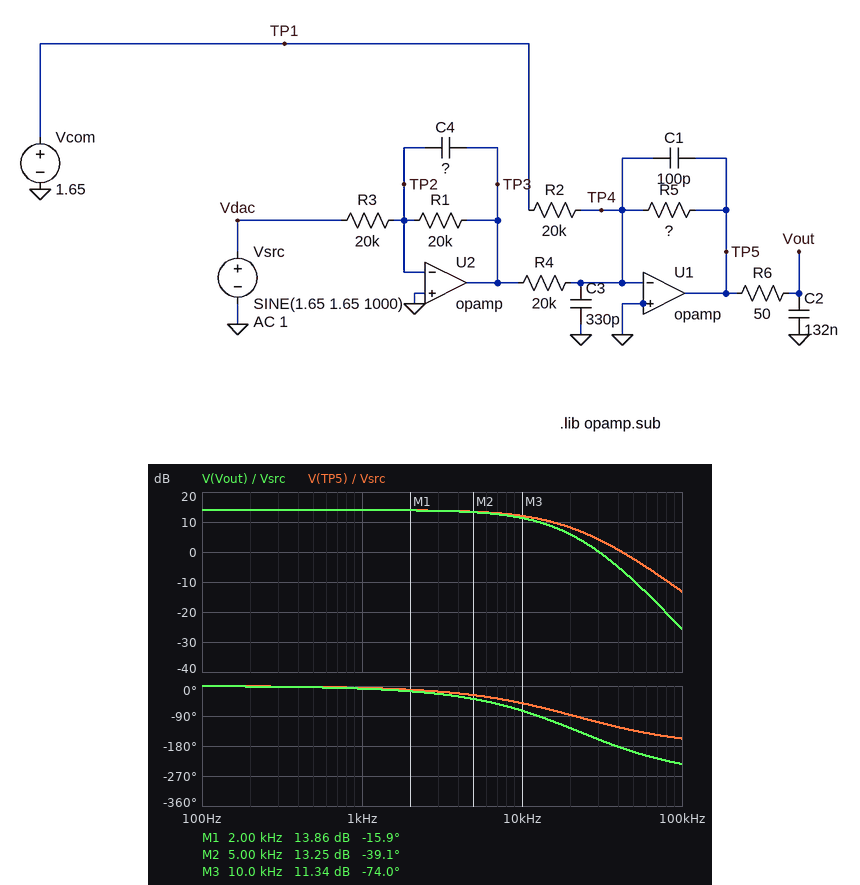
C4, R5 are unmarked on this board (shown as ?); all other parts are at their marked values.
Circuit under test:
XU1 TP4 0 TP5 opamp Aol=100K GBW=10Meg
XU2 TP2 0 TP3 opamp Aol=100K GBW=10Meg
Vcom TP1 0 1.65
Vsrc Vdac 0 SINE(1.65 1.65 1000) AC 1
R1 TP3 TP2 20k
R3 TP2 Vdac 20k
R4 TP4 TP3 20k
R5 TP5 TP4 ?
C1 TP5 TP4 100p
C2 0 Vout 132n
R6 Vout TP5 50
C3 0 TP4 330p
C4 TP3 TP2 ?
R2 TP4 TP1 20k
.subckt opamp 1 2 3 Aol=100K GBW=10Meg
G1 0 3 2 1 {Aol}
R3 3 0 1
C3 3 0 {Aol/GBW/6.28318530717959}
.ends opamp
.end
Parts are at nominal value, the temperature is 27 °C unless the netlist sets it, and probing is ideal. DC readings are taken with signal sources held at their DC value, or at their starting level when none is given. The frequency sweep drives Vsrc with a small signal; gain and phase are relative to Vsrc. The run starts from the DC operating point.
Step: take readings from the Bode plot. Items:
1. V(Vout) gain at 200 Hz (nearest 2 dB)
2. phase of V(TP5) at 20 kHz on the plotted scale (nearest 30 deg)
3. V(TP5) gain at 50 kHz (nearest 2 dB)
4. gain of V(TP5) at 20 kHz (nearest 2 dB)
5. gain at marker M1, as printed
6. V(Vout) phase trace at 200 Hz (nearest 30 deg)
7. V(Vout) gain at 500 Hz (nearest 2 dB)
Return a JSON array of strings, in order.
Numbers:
["14 dB", "-90 deg", "-2 dB", "8 dB", "13.86 dB", "0 deg", "14 dB"]
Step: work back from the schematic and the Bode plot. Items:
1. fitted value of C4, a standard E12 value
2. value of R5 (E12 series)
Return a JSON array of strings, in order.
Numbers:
["270 pF", "100 kΩ"]
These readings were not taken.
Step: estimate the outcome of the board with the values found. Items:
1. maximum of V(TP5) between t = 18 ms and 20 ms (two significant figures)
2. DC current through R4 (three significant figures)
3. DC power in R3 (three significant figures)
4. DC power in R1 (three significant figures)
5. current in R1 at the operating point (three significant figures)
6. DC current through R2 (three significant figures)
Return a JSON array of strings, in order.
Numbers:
["8.2 V", "82.5 µA", "136 µW", "136 µW", "82.5 µA", "82.5 µA"]
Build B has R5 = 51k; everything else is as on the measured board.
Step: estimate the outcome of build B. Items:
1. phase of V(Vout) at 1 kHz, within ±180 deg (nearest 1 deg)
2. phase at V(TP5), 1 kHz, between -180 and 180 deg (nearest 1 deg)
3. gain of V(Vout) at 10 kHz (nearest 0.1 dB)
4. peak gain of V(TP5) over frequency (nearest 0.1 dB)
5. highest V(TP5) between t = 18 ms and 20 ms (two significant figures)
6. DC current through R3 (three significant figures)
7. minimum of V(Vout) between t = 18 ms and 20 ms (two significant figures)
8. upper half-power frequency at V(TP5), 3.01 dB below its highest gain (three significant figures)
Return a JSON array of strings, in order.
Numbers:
["-6 deg", "-4 deg", "6.5 dB", "8.1 dB", "4.2 V", "82.5 µA", "-4.2 V", "19.4 kHz"]
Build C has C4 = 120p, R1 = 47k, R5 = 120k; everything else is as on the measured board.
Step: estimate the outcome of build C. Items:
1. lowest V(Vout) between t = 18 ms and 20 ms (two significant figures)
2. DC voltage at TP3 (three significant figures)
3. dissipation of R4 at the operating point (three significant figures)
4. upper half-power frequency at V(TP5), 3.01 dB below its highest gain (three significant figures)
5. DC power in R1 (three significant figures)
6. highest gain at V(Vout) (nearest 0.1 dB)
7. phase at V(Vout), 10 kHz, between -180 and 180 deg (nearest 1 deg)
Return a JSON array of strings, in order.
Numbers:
["-9.8 V", "-3.88 V", "752 µW", "11.2 kHz", "320 µW", "23.0 dB", "-80 deg"]
